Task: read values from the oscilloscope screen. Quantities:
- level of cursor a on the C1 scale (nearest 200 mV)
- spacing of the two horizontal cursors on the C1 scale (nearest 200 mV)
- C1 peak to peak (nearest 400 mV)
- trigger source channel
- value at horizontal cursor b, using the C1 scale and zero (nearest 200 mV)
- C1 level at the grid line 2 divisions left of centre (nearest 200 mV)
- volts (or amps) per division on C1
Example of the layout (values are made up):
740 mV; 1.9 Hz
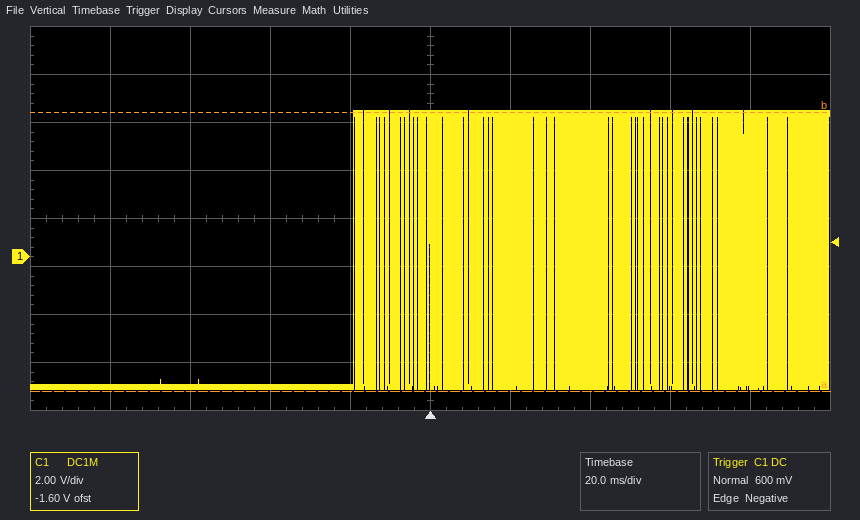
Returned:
-5.6 V; 11.6 V; 11.6 V; C1; 6.0 V; -5.4 V; 2 V
